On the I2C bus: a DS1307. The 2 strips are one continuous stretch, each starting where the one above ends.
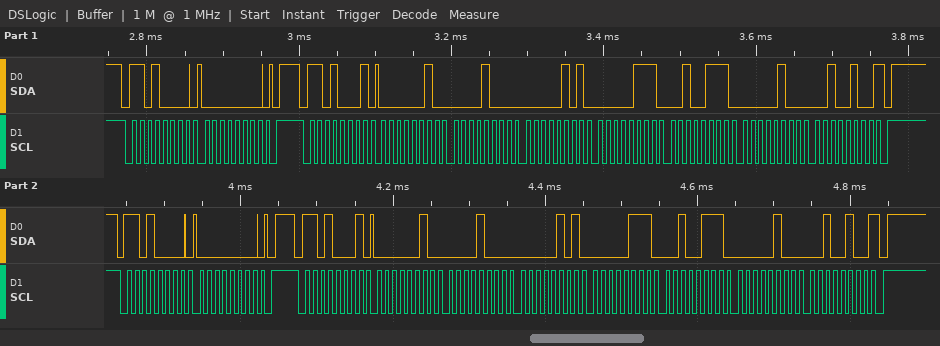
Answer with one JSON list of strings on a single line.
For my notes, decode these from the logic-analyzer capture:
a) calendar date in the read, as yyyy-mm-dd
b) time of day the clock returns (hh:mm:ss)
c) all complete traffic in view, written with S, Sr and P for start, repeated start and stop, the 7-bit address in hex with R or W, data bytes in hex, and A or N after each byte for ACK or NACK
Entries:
["2024-04-27", "05:08:02", "S 68W A 00 A P S 68R A 02 A 08 A 05 A 07 A 27 A 04 A 24 N P S 68W A 00 A P S 68R A 02 A 08 A 05 A 07 A 27 A 04 A 24 N P"]
